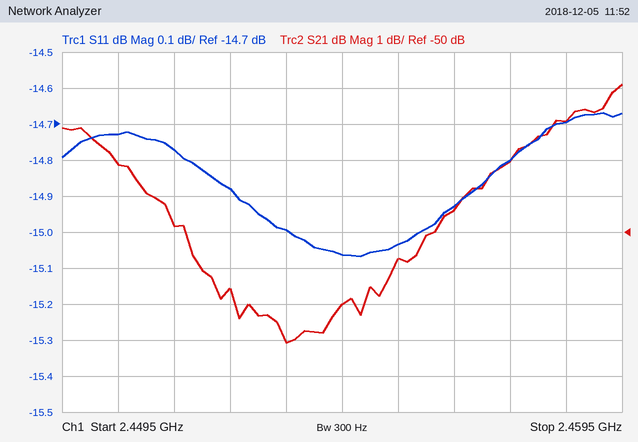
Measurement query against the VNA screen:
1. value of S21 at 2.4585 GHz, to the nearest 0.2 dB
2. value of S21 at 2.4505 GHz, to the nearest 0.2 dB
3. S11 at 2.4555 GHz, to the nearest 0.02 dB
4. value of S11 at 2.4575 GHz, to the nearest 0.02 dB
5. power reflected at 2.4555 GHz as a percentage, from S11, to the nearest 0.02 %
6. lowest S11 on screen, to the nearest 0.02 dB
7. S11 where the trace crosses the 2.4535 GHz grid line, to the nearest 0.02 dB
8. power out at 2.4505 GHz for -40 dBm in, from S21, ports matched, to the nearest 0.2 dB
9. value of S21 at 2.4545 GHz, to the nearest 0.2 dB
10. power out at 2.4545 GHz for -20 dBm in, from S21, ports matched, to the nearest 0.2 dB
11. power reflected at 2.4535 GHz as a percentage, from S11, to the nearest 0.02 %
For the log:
-47.0 dB
-48.2 dB
-15.04 dB
-14.80 dB
3.14 %
-15.06 dB
-15.00 dB
-88.2 dBm
-52.0 dB
-72.0 dBm
3.16 %
